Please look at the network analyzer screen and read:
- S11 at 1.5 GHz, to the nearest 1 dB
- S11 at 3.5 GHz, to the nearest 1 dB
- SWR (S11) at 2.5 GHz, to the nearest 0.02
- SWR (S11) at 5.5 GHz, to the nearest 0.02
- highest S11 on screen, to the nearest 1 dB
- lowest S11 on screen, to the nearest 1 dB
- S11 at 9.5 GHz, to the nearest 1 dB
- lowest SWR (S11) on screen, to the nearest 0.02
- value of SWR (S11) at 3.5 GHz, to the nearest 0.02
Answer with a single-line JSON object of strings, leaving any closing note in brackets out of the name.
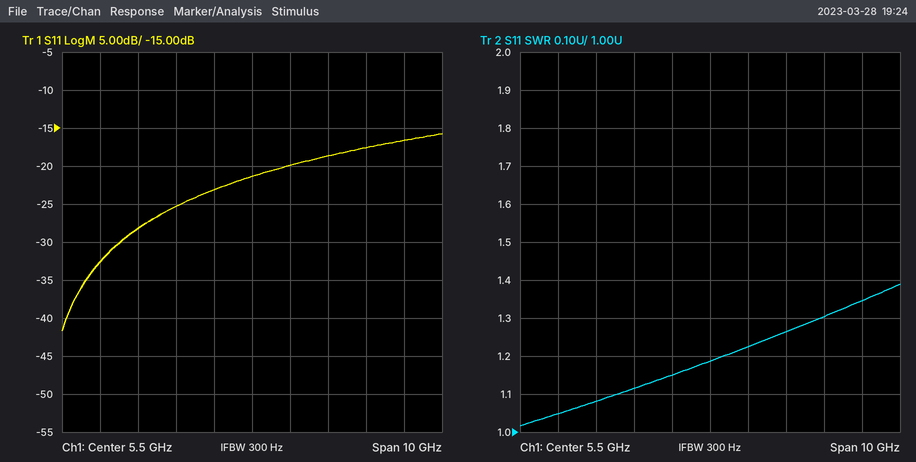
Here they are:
{"S11 at 1.5 GHz, to the nearest 1 dB": "-33 dB", "S11 at 3.5 GHz, to the nearest 1 dB": "-25 dB", "SWR (S11) at 2.5 GHz, to the nearest 0.02": "1.08", "SWR (S11) at 5.5 GHz, to the nearest 0.02": "1.18", "highest S11 on screen, to the nearest 1 dB": "-16 dB", "lowest S11 on screen, to the nearest 1 dB": "-42 dB", "S11 at 9.5 GHz, to the nearest 1 dB": "-17 dB", "lowest SWR (S11) on screen, to the nearest 0.02": "1.02", "value of SWR (S11) at 3.5 GHz, to the nearest 0.02": "1.12"}
